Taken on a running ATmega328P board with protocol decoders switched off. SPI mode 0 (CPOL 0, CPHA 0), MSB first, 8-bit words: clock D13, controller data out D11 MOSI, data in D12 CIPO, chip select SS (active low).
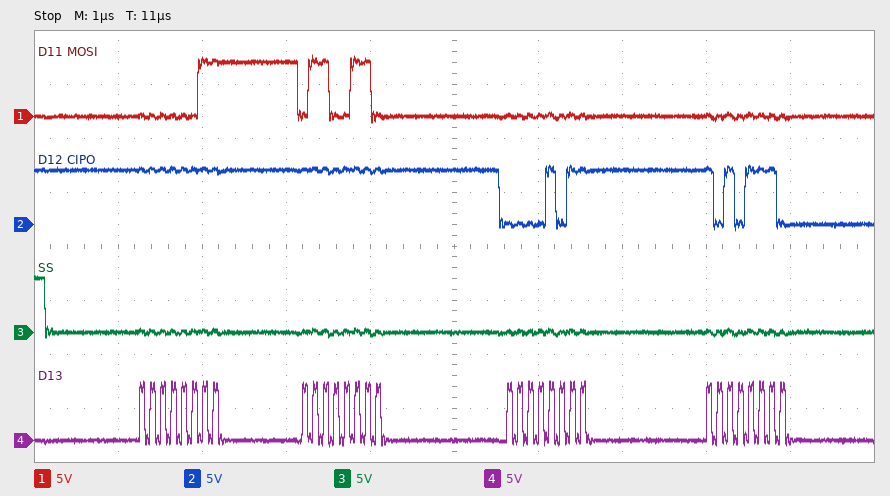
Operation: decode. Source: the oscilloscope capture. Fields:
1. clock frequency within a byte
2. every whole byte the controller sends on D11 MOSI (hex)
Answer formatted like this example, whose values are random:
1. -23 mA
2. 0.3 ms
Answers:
1. 8 MHz
2. 03 66 00 00
